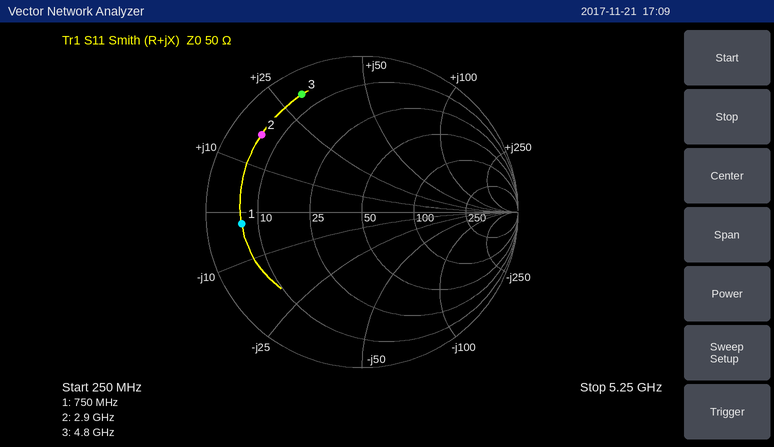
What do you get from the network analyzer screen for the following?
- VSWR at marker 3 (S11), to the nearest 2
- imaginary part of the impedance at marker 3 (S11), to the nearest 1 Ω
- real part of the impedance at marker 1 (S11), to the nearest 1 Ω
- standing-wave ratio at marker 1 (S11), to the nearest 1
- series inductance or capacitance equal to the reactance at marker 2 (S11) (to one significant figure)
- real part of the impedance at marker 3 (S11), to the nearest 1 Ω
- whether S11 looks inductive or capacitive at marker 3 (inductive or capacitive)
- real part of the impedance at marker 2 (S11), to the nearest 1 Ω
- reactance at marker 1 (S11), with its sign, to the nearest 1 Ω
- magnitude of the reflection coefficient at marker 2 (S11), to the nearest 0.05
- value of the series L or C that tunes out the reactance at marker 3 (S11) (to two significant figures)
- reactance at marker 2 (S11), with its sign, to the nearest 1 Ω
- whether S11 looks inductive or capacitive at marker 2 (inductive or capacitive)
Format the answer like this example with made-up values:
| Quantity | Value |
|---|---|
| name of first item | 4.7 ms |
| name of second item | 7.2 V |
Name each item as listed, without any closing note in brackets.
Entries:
| Quantity | Value |
|---|---|
| VSWR at marker 3 (S11), to the nearest 2 | 12 |
| imaginary part of the impedance at marker 3 (S11), to the nearest 1 Ω | +30 Ω |
| real part of the impedance at marker 1 (S11), to the nearest 1 Ω | 6 Ω |
| standing-wave ratio at marker 1 (S11), to the nearest 1 | 8 |
| series inductance or capacitance equal to the reactance at marker 2 (S11) | 900 pH |
| real part of the impedance at marker 3 (S11), to the nearest 1 Ω | 6 Ω |
| whether S11 looks inductive or capacitive at marker 3 | inductive |
| real part of the impedance at marker 2 (S11), to the nearest 1 Ω | 6 Ω |
| reactance at marker 1 (S11), with its sign, to the nearest 1 Ω | -2 Ω |
| magnitude of the reflection coefficient at marker 2 (S11), to the nearest 0.05 | 0.80 |
| value of the series L or C that tunes out the reactance at marker 3 (S11) | 1.1 pF |
| reactance at marker 2 (S11), with its sign, to the nearest 1 Ω | +17 Ω |
| whether S11 looks inductive or capacitive at marker 2 | inductive |
